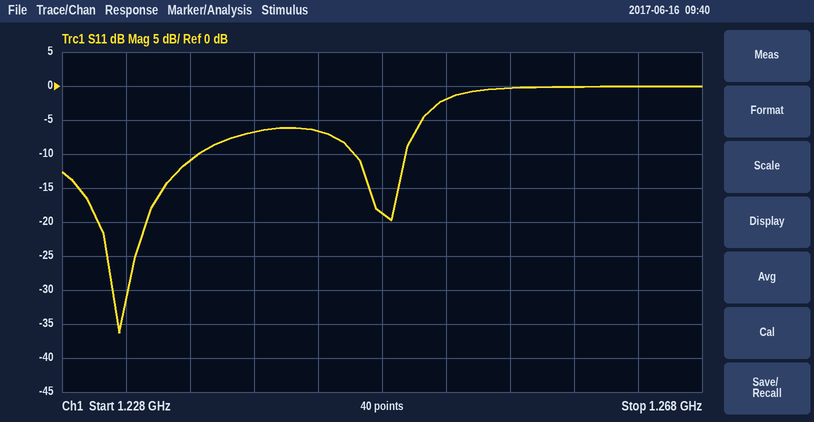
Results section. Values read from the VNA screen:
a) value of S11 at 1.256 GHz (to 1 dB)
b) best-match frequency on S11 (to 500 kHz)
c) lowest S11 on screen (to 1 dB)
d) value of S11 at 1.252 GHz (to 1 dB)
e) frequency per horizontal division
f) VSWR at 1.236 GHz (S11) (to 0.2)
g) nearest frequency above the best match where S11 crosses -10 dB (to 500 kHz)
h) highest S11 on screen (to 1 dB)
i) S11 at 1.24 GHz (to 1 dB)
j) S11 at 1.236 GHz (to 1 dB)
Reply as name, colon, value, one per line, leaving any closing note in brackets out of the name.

value of S11 at 1.256 GHz: 0 dB
best-match frequency on S11: 1.2315 GHz
lowest S11 on screen: -36 dB
value of S11 at 1.252 GHz: -2 dB
frequency per horizontal division: 4 MHz
VSWR at 1.236 GHz (S11): 1.8
nearest frequency above the best match where S11 crosses -10 dB: 1.2365 GHz
highest S11 on screen: 0 dB
S11 at 1.24 GHz: -7 dB
S11 at 1.236 GHz: -11 dB
